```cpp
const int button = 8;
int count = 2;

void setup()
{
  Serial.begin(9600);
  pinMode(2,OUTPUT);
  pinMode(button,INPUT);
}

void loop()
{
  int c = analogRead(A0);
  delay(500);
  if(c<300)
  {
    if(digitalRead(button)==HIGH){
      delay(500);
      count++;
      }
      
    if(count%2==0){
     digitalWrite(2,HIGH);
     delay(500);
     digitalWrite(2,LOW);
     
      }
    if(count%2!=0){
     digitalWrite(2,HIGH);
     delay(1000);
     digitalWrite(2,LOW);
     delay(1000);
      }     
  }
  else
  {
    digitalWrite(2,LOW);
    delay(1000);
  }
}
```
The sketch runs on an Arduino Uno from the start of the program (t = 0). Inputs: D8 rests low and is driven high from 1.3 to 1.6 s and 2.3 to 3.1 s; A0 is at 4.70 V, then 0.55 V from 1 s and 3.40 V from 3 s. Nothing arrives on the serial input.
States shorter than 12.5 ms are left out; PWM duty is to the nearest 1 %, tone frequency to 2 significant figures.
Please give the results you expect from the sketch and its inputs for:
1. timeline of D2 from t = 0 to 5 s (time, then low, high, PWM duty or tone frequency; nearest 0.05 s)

0 s low; 2 s high; 2.5 s low; 3.5 s high; 4.5 s low
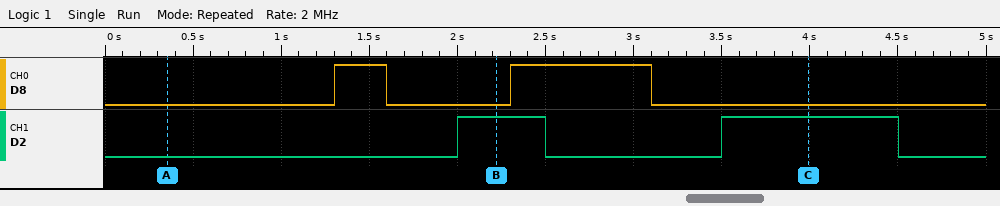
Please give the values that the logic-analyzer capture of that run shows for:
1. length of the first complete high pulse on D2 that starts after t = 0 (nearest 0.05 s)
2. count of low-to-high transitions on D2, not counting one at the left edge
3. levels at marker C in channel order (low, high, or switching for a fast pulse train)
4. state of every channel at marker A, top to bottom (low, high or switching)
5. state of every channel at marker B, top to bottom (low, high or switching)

0.50 s
2
D8 low, D2 high
D8 low, D2 low
D8 low, D2 high
